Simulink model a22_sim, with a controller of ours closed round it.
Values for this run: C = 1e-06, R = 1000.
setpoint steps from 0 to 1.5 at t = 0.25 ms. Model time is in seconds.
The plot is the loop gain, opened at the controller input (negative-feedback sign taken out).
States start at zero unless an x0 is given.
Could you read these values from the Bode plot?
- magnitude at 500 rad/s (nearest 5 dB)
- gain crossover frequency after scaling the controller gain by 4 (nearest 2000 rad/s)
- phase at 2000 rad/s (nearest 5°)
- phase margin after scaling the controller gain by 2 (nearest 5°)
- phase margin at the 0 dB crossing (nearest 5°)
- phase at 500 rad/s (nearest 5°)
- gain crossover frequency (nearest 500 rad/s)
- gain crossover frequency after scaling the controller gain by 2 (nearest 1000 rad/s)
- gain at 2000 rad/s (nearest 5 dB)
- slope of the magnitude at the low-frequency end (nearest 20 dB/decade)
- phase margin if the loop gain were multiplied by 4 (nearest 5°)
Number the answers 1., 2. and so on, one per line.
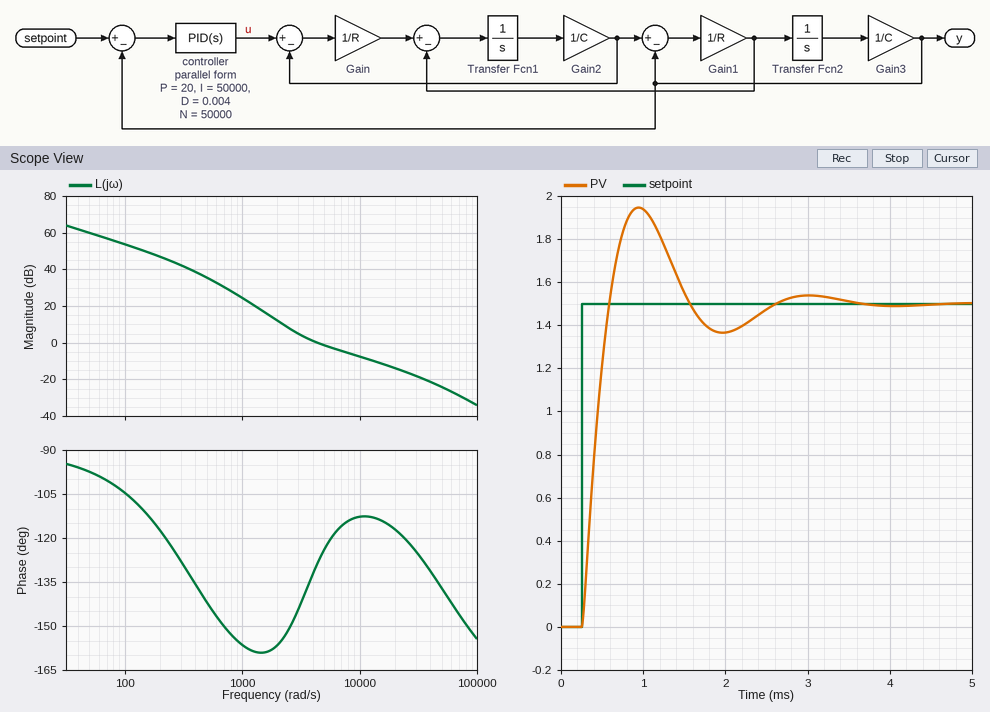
1. 35 dB
2. 16000 rad/s
3. -155°
4. 65°
5. 50°
6. -140°
7. 4500 rad/s
8. 8000 rad/s
9. 10 dB
10. -20 dB/decade
11. 65°
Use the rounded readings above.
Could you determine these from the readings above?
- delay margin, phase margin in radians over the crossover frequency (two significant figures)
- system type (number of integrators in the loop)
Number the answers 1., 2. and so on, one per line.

1. 0.00019 s
2. 1
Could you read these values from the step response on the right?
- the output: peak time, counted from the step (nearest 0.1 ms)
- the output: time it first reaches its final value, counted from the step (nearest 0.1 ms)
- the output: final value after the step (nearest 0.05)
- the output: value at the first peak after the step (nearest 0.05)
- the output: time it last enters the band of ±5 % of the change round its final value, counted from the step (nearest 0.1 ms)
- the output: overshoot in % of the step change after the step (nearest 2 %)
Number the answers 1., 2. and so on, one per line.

1. 0.7 ms
2. 0.3 ms
3. 1.50
4. 1.95
5. 2.1 ms
6. 30 %
